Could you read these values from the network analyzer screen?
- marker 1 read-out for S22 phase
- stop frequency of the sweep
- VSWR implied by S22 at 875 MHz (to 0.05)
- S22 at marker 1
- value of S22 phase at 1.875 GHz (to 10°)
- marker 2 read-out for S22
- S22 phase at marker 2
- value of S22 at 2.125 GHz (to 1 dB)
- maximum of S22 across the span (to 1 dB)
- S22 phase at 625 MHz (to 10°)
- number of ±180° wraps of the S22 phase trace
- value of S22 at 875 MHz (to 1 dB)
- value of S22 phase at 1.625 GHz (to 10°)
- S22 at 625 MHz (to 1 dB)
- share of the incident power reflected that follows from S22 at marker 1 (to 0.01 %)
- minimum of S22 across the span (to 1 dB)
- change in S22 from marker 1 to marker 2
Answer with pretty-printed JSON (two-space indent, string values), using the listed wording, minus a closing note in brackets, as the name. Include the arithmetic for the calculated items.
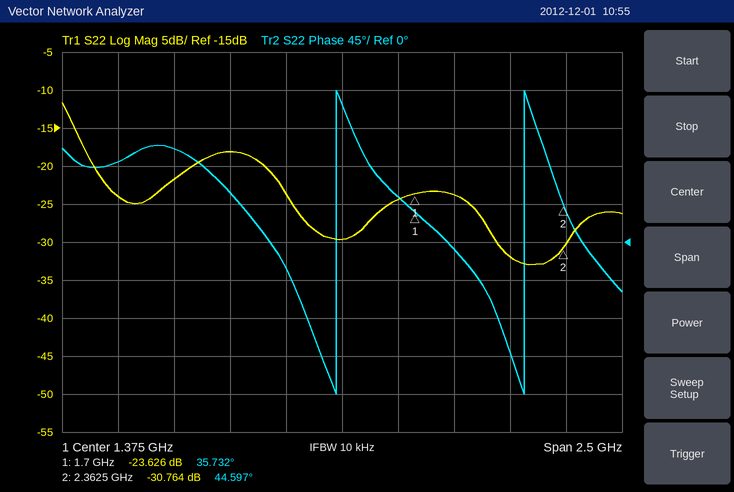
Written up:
{
  "marker 1 read-out for S22 phase": "35.732°",
  "stop frequency of the sweep": "2.625 GHz",
  "VSWR implied by S22 at 875 MHz": "|Γ| = 10^(-18/20) = 0.1259; VSWR = (1 + 0.1259)/(1 − 0.1259) ≈ 1.29, so 1.30 to the nearest 0.05",
  "S22 at marker 1": "-23.626 dB",
  "value of S22 phase at 1.875 GHz": "-10°",
  "marker 2 read-out for S22": "-30.764 dB",
  "S22 phase at marker 2": "44.597°",
  "value of S22 at 2.125 GHz": "-32 dB",
  "maximum of S22 across the span": "-12 dB",
  "S22 phase at 625 MHz": "110°",
  "number of ±180° wraps of the S22 phase trace": "2",
  "value of S22 at 875 MHz": "-18 dB",
  "value of S22 phase at 1.625 GHz": "50°",
  "S22 at 625 MHz": "-22 dB",
  "share of the incident power reflected that follows from S22 at marker 1": "10^(-23.626/10) ≈ 0.43 %",
  "minimum of S22 across the span": "-33 dB",
  "change in S22 from marker 1 to marker 2": "-30.764 − (-23.626) = -7.138 dB"
}
